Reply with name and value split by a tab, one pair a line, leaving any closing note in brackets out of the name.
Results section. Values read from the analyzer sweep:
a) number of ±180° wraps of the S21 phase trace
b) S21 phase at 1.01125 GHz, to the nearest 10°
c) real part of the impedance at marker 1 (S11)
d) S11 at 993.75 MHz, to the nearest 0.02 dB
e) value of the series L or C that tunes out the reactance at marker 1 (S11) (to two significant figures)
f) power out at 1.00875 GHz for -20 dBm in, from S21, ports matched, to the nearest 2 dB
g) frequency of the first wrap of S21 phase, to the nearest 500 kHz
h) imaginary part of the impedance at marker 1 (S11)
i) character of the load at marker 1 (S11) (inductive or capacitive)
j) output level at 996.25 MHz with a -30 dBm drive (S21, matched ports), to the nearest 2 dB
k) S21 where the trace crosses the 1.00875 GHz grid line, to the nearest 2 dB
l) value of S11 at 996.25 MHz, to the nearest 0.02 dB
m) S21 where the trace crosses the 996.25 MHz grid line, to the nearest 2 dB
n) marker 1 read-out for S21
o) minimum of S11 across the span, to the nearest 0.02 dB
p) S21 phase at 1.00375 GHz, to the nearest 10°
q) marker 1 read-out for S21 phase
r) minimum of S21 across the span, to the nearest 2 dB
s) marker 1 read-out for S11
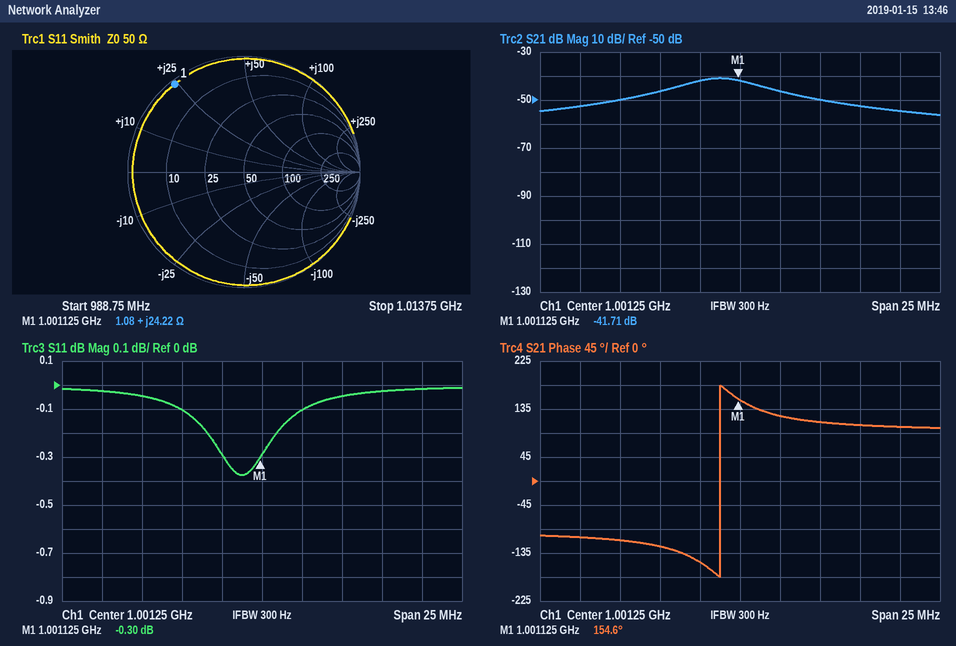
number of ±180° wraps of the S21 phase trace	1
S21 phase at 1.01125 GHz, to the nearest 10°	100°
real part of the impedance at marker 1	1.08 Ω
S11 at 993.75 MHz, to the nearest 0.02 dB	-0.04 dB
value of the series L or C that tunes out the reactance at marker 1 (S11)	6.6 pF
power out at 1.00875 GHz for -20 dBm in, from S21, ports matched, to the nearest 2 dB	-72 dBm
frequency of the first wrap of S21 phase, to the nearest 500 kHz	1.0000 GHz
imaginary part of the impedance at marker 1	+24.22 Ω
character of the load at marker 1 (S11)	inductive
output level at 996.25 MHz with a -30 dBm drive (S21, matched ports), to the nearest 2 dB	-76 dBm
S21 where the trace crosses the 1.00875 GHz grid line, to the nearest 2 dB	-52 dB
value of S11 at 996.25 MHz, to the nearest 0.02 dB	-0.10 dB
S21 where the trace crosses the 996.25 MHz grid line, to the nearest 2 dB	-46 dB
marker 1 read-out for S21	-41.71 dB
minimum of S11 across the span, to the nearest 0.02 dB	-0.38 dB
S21 phase at 1.00375 GHz, to the nearest 10°	120°
marker 1 read-out for S21 phase	154.6°
minimum of S21 across the span, to the nearest 2 dB	-56 dB
marker 1 read-out for S11	-0.30 dB
